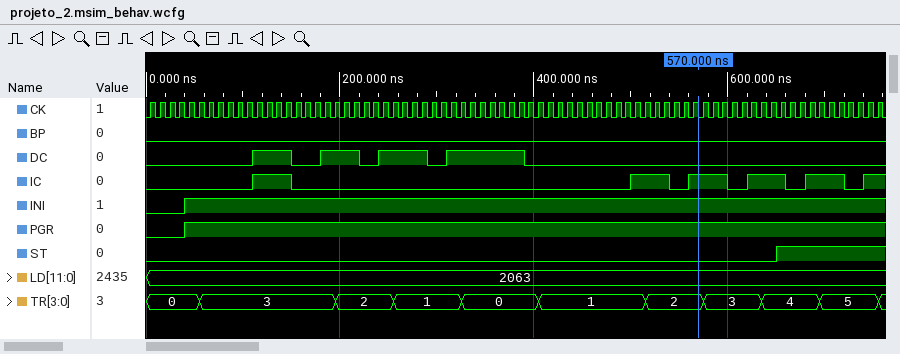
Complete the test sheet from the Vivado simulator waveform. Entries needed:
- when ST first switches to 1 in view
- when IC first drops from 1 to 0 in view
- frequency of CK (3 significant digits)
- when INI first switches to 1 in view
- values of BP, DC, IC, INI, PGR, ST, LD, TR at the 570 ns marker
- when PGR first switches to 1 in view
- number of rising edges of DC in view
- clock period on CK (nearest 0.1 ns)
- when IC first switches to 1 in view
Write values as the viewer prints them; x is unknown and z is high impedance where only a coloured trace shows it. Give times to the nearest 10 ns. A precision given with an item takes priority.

650 ns
150 ns
100 MHz
40 ns
BP=0, DC=0, IC=1, INI=1, PGR=1, ST=0, LD=2063, TR=2
40 ns
4
10 ns
110 ns
